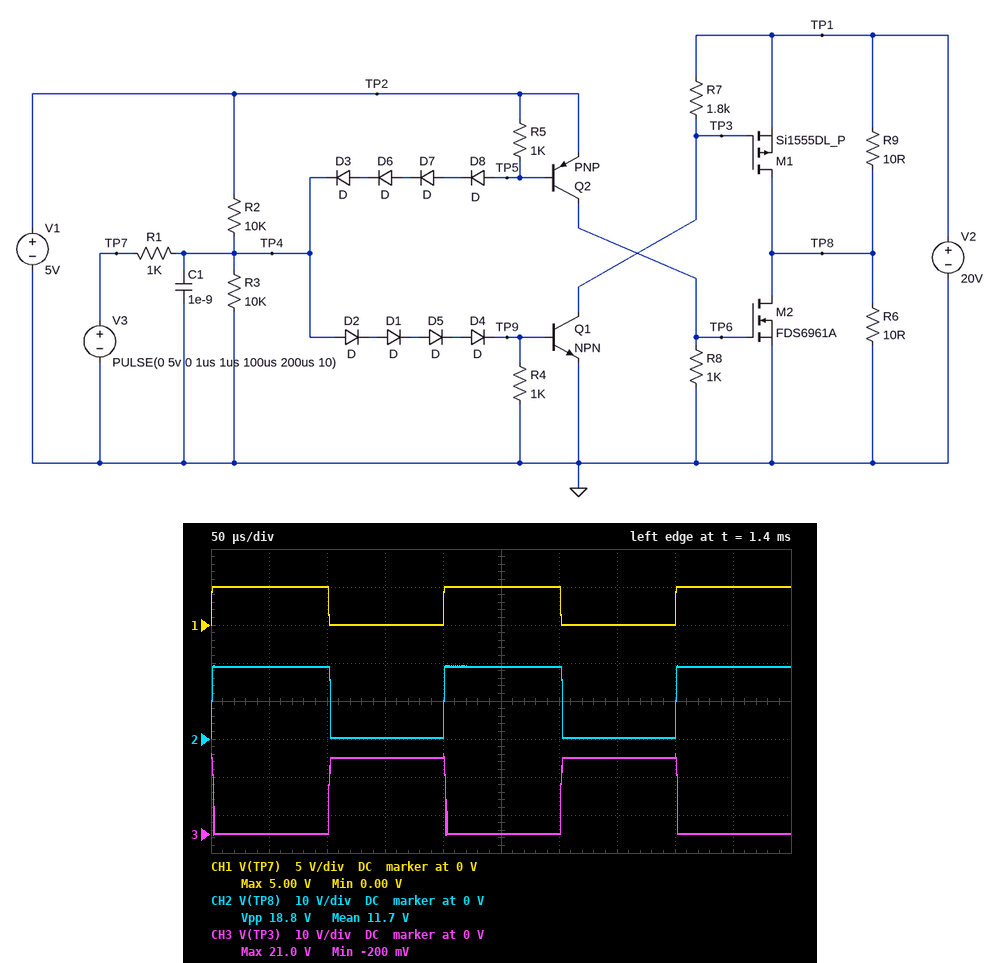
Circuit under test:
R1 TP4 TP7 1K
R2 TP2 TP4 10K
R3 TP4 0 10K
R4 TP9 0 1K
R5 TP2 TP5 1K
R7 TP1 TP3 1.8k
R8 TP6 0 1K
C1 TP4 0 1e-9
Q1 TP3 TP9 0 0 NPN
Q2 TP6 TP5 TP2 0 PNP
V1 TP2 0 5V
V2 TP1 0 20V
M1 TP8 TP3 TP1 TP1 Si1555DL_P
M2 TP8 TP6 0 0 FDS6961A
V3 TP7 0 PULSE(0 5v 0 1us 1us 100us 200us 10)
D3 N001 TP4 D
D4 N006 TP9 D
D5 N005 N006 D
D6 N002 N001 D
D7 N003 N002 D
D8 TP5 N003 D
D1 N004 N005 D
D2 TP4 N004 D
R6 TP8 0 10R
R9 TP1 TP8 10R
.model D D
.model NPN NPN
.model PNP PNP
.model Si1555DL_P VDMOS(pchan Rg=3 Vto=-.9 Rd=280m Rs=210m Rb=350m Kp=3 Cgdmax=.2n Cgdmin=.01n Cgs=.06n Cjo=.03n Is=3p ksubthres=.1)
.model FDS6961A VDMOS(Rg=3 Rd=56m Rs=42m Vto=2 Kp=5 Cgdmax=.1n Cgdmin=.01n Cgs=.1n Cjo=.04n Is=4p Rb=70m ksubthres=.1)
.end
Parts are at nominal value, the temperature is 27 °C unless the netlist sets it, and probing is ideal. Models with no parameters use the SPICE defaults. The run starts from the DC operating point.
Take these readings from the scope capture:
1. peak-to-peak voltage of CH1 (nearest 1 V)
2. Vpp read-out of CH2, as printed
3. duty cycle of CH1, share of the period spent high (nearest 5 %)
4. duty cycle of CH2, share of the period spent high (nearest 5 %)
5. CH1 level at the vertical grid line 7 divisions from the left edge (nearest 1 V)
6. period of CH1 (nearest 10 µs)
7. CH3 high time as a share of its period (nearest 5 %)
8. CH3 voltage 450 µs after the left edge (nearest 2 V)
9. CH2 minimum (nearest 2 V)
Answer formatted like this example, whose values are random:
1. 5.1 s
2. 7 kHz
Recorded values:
1. 5 V
2. 18.8 V
3. 50 %
4. 50 %
5. 0 V
6. 200 µs
7. 50 %
8. 0 V
9. 0 V
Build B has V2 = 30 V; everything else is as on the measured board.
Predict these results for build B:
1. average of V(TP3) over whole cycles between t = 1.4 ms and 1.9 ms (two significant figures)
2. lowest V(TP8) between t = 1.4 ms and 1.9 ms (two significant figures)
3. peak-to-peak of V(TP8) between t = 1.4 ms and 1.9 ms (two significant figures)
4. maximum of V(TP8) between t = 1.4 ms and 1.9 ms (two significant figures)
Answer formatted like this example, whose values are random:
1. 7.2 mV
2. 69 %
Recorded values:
1. 15 V
2. 500 mV
3. 28 V
4. 29 V
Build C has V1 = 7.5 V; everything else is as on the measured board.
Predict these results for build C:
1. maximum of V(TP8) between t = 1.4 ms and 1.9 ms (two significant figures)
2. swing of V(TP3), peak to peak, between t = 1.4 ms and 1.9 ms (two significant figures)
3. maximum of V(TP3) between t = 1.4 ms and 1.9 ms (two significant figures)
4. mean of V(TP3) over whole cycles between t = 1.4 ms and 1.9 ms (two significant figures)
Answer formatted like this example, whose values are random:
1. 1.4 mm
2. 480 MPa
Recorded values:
1. 4.8 V
2. 1.8 mV
3. 29 mV
4. 28 mV
